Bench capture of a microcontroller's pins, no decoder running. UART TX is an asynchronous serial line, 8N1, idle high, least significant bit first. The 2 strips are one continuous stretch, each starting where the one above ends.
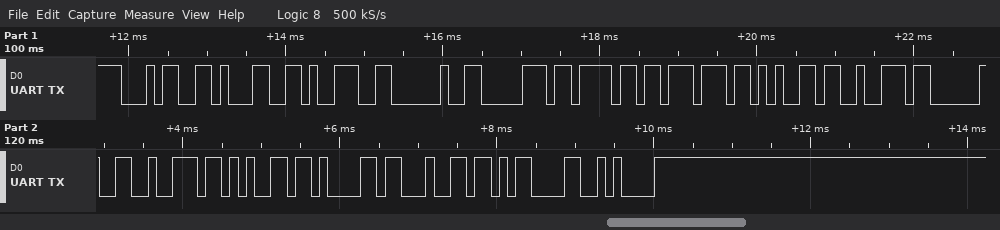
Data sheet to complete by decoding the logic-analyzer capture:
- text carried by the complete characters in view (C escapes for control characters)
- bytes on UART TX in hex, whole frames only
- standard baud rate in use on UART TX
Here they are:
"419 power read\r\n"
34 31 39 20 70 6F 77 65 72 20 72 65 61 64 0D 0A
9600 baud
